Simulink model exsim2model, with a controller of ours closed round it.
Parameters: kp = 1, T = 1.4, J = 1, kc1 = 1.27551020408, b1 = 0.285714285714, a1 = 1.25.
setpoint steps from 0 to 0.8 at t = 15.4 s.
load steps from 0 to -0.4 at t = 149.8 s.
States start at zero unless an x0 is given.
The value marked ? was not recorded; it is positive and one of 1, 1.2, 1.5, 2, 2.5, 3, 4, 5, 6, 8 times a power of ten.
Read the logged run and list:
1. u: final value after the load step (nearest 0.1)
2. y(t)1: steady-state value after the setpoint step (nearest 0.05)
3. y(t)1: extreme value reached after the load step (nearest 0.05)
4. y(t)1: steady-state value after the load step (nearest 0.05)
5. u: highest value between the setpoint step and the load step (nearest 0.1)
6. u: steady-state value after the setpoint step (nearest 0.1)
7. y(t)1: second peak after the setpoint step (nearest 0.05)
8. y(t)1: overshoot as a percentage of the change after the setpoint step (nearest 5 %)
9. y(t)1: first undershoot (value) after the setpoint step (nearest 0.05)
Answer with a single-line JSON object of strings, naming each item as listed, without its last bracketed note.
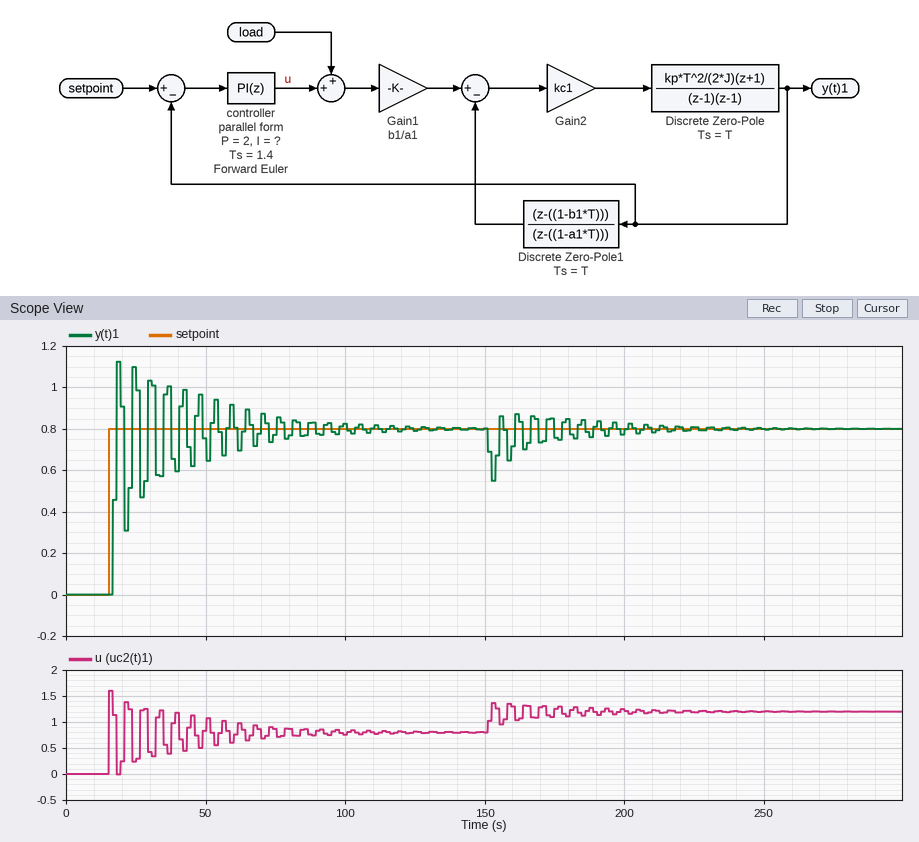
{"u: final value after the load step": "1.2", "y(t)1: steady-state value after the setpoint step": "0.80", "y(t)1: extreme value reached after the load step": "0.55", "y(t)1: steady-state value after the load step": "0.80", "u: highest value between the setpoint step and the load step": "1.6", "u: steady-state value after the setpoint step": "0.8", "y(t)1: second peak after the setpoint step": "1.10", "y(t)1: overshoot as a percentage of the change after the setpoint step": "40 %", "y(t)1: first undershoot (value) after the setpoint step": "0.30"}
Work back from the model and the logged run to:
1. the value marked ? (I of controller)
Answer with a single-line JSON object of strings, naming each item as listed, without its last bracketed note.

{"the value marked ?": "0.4"}
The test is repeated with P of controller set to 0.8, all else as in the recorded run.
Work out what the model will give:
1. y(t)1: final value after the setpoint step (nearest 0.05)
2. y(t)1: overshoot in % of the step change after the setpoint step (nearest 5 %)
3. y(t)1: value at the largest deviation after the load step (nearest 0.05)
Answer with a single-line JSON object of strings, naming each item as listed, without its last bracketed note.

{"y(t)1: final value after the setpoint step": "0.80", "y(t)1: overshoot in % of the step change after the setpoint step": "15 %", "y(t)1: value at the largest deviation after the load step": "0.50"}
